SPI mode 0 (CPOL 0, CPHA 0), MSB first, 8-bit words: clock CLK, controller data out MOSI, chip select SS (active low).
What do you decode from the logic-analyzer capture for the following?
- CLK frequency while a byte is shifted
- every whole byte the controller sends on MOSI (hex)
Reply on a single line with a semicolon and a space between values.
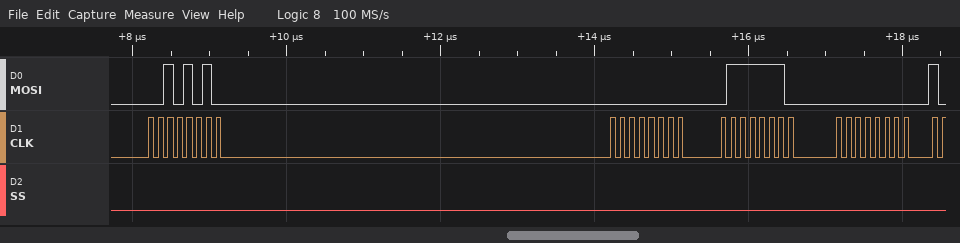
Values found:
8 MHz; 0x2A 0x00 0x7E 0x00
